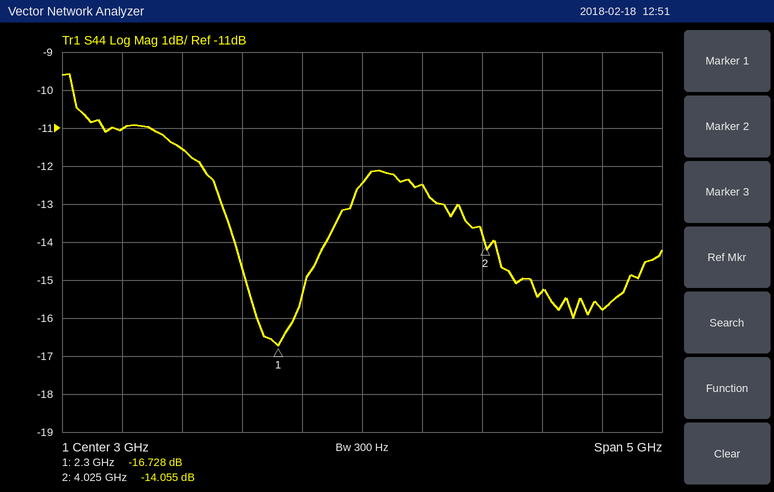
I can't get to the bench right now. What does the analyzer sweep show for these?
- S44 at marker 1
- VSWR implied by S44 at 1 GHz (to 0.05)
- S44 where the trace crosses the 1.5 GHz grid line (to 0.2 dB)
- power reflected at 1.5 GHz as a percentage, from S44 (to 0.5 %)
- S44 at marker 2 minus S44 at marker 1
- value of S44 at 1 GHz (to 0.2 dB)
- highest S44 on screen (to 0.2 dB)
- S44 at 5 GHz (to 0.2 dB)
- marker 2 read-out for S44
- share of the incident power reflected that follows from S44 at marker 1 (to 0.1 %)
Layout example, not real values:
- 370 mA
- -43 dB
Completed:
- -16.728 dB
- 1.80
- -11.6 dB
- 7.0 %
- 2.673 dB
- -11.0 dB
- -9.6 dB
- -15.8 dB
- -14.055 dB
- 2.1 %
